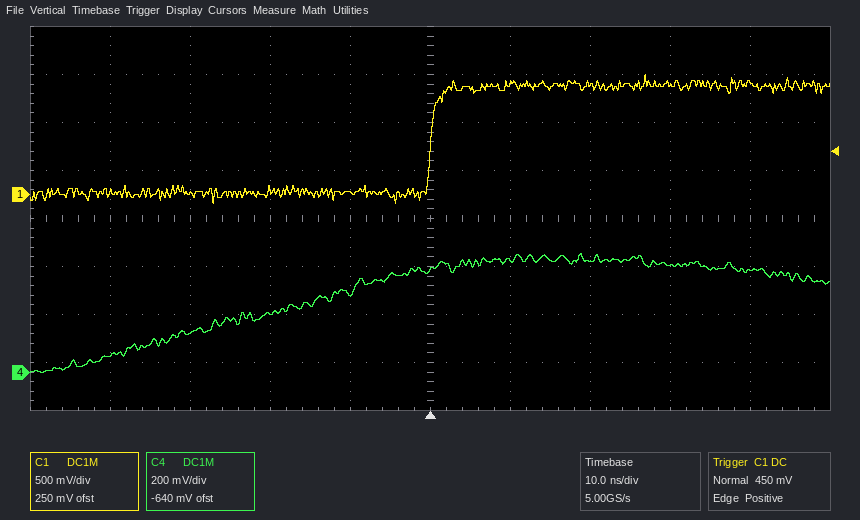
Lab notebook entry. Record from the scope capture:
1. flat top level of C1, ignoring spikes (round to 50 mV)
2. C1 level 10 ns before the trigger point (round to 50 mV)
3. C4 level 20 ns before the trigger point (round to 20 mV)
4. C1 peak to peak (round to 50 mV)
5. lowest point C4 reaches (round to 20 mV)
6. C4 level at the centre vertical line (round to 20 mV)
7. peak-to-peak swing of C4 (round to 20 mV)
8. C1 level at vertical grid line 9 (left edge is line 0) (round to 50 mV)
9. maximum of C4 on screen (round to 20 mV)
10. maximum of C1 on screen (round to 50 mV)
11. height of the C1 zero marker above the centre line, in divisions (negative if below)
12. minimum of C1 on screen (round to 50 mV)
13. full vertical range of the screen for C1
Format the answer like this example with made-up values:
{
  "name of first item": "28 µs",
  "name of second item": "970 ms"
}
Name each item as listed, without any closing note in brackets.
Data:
{
  "flat top level of C1, ignoring spikes": "1.15 V",
  "C1 level 10 ns before the trigger point": "0 mV",
  "C4 level 20 ns before the trigger point": "240 mV",
  "C1 peak to peak": "1.35 V",
  "lowest point C4 reaches": "0 mV",
  "C4 level at the centre vertical line": "420 mV",
  "peak-to-peak swing of C4": "500 mV",
  "C1 level at vertical grid line 9 (left edge is line 0)": "1.15 V",
  "maximum of C4 on screen": "500 mV",
  "maximum of C1 on screen": "1.25 V",
  "height of the C1 zero marker above the centre line, in divisions": "+0.5 div",
  "minimum of C1 on screen": "-100 mV",
  "full vertical range of the screen for C1": "4 V"
}
